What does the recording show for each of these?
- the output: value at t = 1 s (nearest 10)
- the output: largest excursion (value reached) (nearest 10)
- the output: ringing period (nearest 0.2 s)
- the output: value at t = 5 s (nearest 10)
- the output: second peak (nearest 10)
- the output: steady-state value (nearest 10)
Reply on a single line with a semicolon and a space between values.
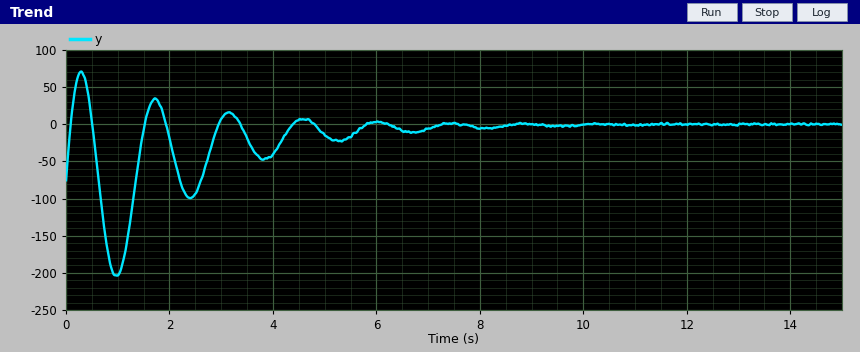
-200; 70; 1.4 s; -10; 30; 0
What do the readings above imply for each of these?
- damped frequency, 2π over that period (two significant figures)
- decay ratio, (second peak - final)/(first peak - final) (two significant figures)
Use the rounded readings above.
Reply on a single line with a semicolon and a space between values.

4.5 rad/s; 0.43
